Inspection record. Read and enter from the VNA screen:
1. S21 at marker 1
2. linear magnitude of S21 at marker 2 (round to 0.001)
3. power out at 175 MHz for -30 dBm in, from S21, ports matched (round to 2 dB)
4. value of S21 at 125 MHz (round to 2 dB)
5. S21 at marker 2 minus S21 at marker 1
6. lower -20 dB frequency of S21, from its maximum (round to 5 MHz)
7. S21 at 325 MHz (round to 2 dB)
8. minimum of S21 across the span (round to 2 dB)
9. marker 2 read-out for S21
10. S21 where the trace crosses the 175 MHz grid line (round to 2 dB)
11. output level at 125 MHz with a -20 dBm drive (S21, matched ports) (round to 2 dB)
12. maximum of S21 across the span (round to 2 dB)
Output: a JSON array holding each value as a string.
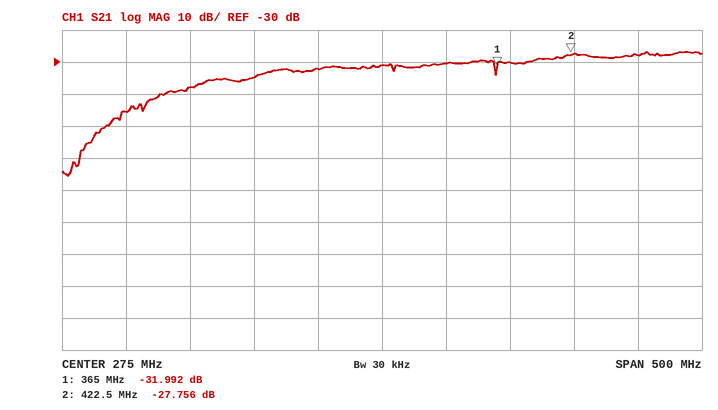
["-31.992 dB", "0.041", "-64 dBm", "-38 dB", "4.236 dB", "70 MHz", "-30 dB", "-66 dB", "-27.756 dB", "-34 dB", "-58 dBm", "-26 dB"]
